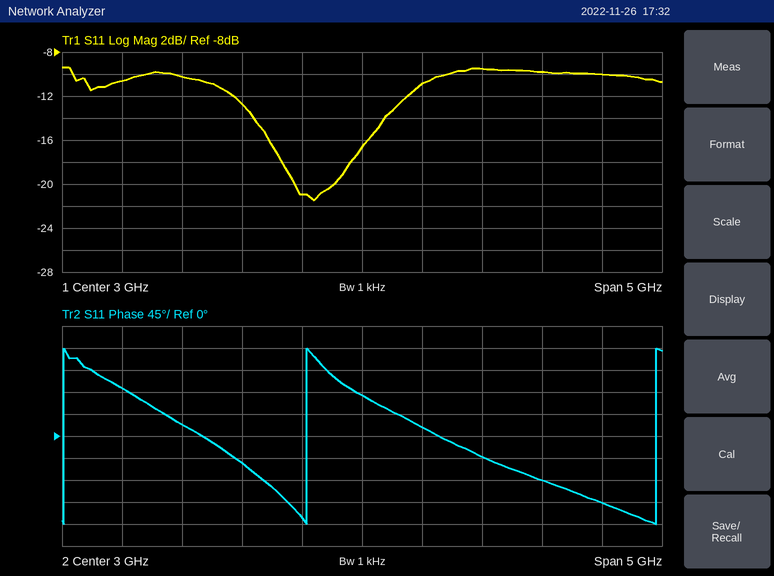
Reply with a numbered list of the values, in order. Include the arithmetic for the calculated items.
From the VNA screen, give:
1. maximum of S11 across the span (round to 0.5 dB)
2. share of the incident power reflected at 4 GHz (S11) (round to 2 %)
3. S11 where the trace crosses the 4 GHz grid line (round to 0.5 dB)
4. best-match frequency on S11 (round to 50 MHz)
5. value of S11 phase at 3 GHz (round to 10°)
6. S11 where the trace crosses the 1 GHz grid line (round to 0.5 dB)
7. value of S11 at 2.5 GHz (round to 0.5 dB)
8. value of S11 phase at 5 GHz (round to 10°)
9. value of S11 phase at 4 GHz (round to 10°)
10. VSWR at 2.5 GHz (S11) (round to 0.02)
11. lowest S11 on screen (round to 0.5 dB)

1. -9.5 dB
2. 10^(-9.5/10) ≈ 11.2 %, so 12 % to the nearest 2 %
3. -9.5 dB
4. 2.60 GHz
5. 80°
6. -10.5 dB
7. -21.0 dB
8. -140°
9. -40°
10. |Γ| = 10^(-21/20) = 0.0891; VSWR = (1 + 0.0891)/(1 − 0.0891) ≈ 1.20
11. -21.5 dB
